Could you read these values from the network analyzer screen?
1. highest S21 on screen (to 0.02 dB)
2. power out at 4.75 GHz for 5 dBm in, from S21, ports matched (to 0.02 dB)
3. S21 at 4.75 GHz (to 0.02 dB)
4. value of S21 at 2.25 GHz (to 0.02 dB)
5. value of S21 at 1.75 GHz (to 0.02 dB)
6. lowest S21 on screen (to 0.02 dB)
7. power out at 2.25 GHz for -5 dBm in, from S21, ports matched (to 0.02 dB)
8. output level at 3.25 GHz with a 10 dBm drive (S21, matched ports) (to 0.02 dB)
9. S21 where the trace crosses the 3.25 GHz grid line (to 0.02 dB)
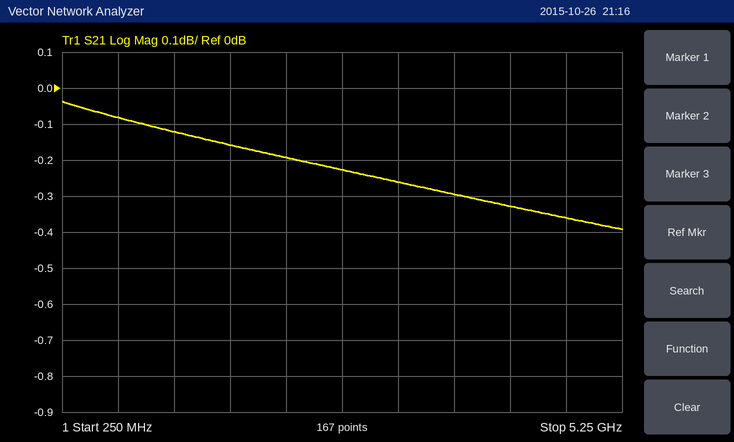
-0.04 dB
4.64 dBm
-0.36 dB
-0.20 dB
-0.16 dB
-0.40 dB
-5.20 dBm
9.74 dBm
-0.26 dB
